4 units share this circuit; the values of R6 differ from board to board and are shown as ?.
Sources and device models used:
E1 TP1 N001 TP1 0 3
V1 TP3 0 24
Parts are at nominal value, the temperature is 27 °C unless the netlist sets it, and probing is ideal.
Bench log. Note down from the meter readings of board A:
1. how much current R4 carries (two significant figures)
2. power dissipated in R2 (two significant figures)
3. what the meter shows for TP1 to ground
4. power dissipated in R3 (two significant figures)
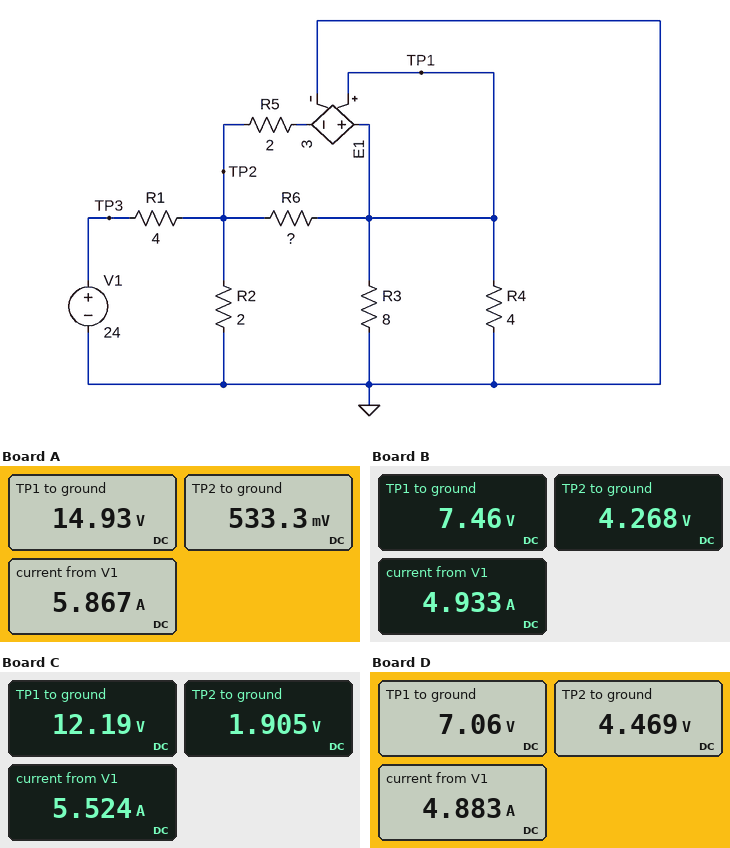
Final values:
3.7 A
140 mW
14.93 V
28 W
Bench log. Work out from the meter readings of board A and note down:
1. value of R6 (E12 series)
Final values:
1.5 Ω
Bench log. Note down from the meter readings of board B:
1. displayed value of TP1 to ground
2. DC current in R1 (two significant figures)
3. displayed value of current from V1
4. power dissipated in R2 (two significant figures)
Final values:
7.46 V
4.9 A
4.933 A
9.1 W
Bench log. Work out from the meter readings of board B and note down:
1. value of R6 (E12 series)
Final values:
0.47 Ω
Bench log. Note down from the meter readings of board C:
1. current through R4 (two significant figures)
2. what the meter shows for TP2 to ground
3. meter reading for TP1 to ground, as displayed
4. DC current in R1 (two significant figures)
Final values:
3.0 A
1.905 V
12.19 V
5.5 A
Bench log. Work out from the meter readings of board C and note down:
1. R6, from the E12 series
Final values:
1.2 Ω
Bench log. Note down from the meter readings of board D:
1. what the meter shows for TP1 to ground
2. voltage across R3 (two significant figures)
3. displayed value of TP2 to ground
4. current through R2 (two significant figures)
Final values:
7.06 V
7.1 V
4.469 V
2.2 A
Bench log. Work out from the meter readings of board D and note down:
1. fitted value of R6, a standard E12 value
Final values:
0.39 Ω
